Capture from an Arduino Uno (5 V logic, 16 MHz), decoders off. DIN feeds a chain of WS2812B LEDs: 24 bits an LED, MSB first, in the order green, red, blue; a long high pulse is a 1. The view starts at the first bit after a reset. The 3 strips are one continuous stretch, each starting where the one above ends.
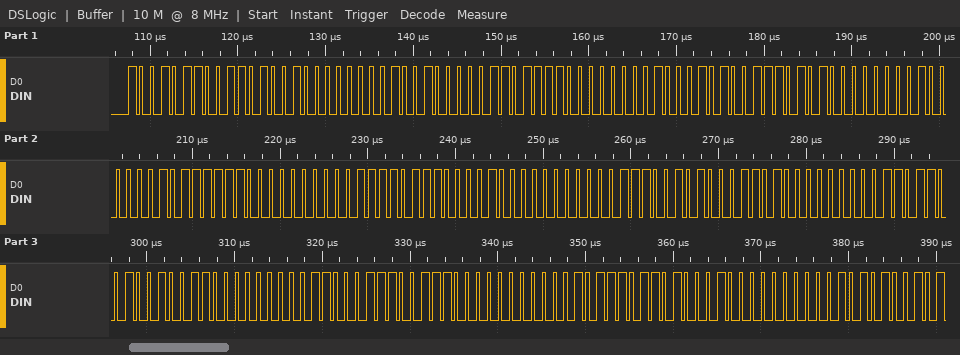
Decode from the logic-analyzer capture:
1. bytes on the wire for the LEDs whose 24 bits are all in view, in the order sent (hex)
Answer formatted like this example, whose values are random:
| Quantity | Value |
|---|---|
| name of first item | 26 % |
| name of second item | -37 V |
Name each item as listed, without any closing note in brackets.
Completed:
| Quantity | Value |
|---|---|
| bytes on the wire for the LEDs whose 24 bits are all in view, in the order sent | 96 69 00 90 6F 00 8A 75 00 81 7E 00 7B 84 00 72 8D 00 6C 93 00 63 9C 00 5D A2 00 |
